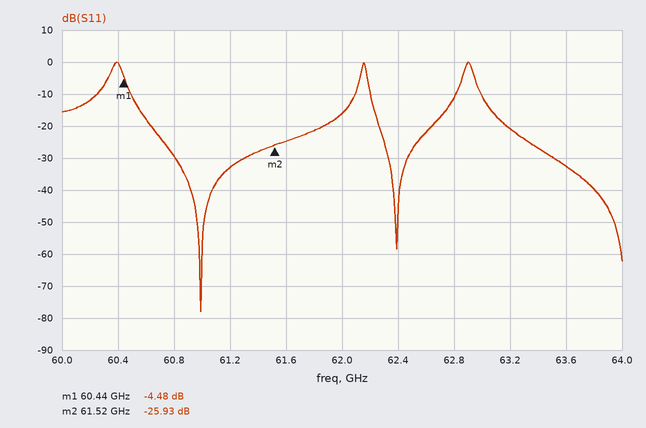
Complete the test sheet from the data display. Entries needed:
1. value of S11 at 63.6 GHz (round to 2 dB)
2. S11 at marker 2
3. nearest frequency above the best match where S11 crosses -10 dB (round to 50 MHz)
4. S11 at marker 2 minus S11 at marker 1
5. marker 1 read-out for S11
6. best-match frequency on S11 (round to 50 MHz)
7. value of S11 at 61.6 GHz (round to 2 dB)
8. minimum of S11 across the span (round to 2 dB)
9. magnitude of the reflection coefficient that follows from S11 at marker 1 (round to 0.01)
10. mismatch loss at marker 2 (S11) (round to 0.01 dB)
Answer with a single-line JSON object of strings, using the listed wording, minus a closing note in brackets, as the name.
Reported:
{"value of S11 at 63.6 GHz": "-32 dB", "S11 at marker 2": "-25.93 dB", "nearest frequency above the best match where S11 crosses -10 dB": "62.10 GHz", "S11 at marker 2 minus S11 at marker 1": "-21.45 dB", "marker 1 read-out for S11": "-4.48 dB", "best-match frequency on S11": "61.00 GHz", "value of S11 at 61.6 GHz": "-24 dB", "minimum of S11 across the span": "-78 dB", "magnitude of the reflection coefficient that follows from S11 at marker 1": "0.60", "mismatch loss at marker 2 (S11)": "0.01 dB"}
